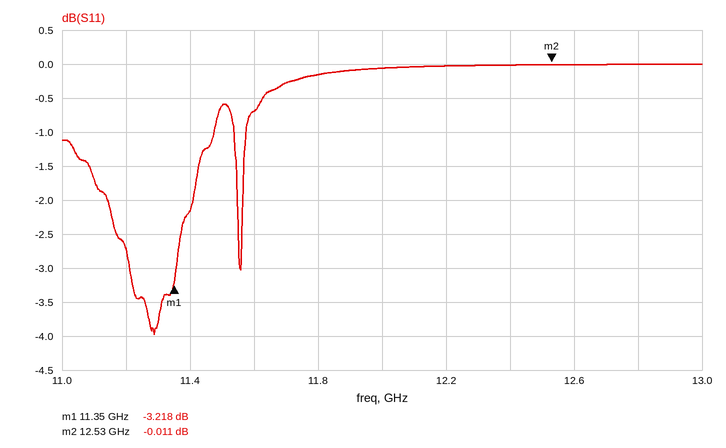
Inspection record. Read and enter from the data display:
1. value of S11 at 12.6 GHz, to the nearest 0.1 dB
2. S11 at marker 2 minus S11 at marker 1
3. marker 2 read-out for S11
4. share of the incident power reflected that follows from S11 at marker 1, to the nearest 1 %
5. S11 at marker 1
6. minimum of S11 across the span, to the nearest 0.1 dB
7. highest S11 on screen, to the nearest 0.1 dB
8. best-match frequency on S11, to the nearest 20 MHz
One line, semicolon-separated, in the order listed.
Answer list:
0.0 dB; 3.207 dB; -0.011 dB; 48 %; -3.218 dB; -4.0 dB; 0.0 dB; 11.28 GHz
